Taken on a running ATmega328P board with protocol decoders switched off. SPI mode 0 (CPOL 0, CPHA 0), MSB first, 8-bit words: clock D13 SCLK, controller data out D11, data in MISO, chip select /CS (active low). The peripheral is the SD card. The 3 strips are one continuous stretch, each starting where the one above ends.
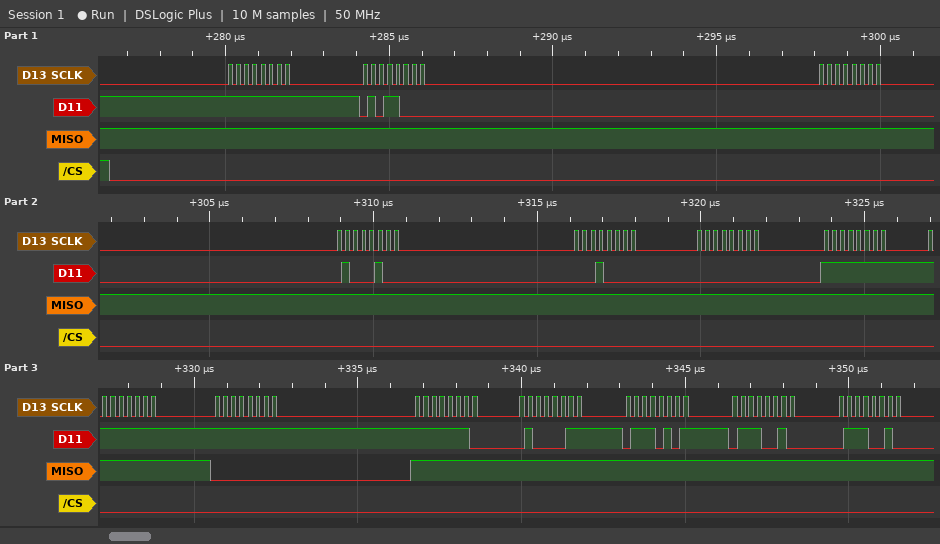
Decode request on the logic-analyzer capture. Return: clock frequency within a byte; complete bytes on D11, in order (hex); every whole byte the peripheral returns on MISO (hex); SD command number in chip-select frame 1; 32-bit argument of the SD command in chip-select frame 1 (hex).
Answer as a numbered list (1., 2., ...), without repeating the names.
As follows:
1. 4 MHz
2. FF 58 00 44 10 00 FF FF FF FE 43 75 72 72
3. FF FF FF FF FF FF FF FF 00 FF FF FF FF FF
4. CMD24
5. 0x00441000
